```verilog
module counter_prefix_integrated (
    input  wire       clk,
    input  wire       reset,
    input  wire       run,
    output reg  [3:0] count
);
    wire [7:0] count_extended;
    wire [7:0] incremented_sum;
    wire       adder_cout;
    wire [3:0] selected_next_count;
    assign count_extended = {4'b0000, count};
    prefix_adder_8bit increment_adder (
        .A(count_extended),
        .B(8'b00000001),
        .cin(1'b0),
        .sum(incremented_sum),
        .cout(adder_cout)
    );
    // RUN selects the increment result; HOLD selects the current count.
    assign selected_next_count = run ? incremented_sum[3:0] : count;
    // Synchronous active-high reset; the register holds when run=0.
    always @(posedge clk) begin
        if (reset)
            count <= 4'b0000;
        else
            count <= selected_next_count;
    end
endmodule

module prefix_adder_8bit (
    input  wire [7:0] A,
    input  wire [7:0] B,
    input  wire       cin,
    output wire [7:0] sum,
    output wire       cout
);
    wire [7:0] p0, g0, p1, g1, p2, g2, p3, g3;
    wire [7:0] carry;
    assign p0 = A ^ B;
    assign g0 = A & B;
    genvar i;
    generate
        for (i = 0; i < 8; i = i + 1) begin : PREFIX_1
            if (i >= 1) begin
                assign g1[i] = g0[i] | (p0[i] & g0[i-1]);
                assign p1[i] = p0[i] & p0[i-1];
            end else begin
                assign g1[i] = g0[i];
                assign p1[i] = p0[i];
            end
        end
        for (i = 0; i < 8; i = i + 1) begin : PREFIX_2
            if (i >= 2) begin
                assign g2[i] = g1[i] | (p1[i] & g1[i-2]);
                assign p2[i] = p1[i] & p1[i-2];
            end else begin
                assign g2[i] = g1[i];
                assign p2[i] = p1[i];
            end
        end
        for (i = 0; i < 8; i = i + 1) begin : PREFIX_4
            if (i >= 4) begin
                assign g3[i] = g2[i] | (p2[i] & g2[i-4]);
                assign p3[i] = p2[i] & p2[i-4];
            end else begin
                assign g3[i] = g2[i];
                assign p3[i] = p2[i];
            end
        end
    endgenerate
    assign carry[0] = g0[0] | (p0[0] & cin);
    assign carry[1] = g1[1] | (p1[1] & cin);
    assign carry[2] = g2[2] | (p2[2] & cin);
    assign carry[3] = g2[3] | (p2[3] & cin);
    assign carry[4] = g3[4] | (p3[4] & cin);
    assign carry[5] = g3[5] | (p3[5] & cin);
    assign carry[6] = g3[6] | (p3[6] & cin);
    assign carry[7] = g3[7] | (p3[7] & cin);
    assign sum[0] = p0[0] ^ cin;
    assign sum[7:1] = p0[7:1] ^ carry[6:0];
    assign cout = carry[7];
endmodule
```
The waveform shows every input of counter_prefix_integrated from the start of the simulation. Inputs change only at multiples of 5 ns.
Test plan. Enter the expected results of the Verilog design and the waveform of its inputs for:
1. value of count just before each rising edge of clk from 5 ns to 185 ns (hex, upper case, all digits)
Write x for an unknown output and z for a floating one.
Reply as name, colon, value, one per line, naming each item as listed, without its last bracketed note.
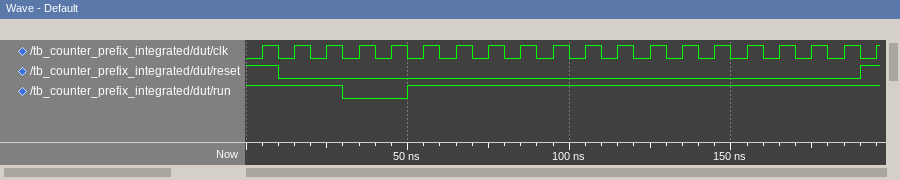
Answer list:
value of count just before each rising edge of clk from 5 ns to 185 ns: x, 0, 1, 2, 2, 2, 3, 4, 5, 6, 7, 8, 9, A, B, C, D, E, F
